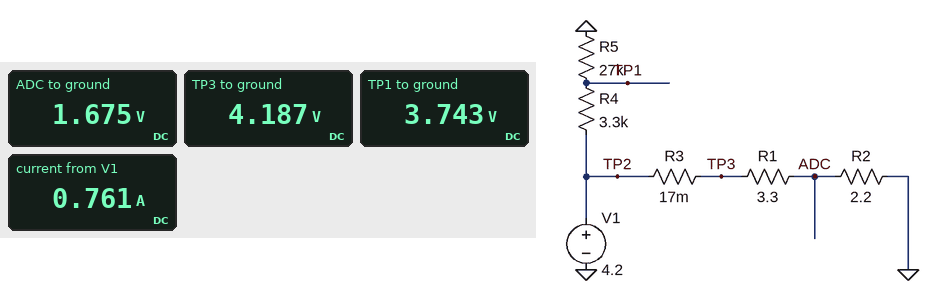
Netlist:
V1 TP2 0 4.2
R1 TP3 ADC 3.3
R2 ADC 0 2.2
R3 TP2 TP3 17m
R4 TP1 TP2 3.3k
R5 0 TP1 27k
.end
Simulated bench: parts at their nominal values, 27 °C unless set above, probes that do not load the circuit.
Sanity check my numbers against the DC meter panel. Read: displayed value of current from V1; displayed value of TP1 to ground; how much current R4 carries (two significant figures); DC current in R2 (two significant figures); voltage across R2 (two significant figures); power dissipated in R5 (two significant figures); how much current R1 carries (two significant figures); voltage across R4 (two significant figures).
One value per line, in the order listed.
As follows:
0.761 A
3.743 V
140 µA
760 mA
1.7 V
520 µW
760 mA
460 mV
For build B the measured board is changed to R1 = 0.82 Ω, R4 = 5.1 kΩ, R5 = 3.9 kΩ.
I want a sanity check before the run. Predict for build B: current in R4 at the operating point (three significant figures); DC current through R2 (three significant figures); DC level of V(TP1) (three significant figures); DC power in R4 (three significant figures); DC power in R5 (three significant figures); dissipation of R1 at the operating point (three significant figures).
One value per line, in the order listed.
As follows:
467 µA
1.38 A
1.82 V
1.11 mW
849 µW
1.57 W
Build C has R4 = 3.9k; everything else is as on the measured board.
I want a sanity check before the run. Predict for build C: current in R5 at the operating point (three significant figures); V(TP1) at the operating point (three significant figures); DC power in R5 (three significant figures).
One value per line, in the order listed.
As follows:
136 µA
3.67 V
499 µW
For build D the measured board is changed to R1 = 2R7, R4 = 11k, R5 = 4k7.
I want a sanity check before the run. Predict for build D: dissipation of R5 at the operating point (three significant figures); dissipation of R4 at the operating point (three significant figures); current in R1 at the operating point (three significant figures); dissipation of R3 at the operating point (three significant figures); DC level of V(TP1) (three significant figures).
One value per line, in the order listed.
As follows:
336 µW
787 µW
854 mA
12.4 mW
1.26 V
